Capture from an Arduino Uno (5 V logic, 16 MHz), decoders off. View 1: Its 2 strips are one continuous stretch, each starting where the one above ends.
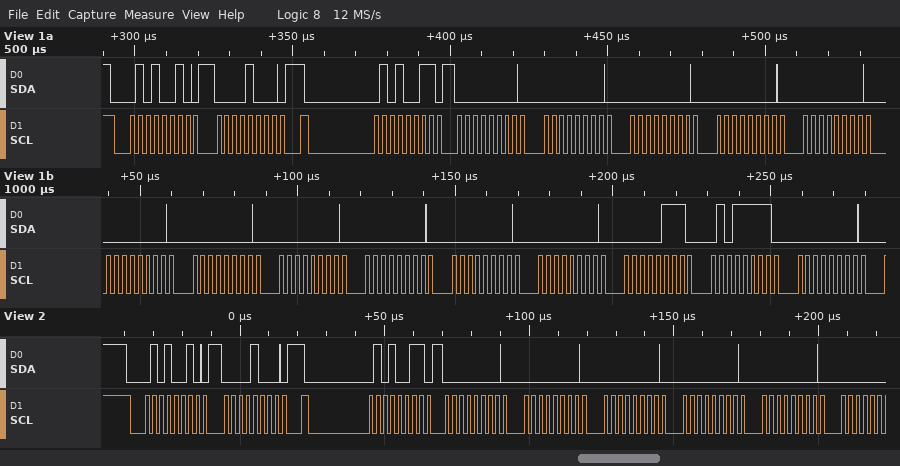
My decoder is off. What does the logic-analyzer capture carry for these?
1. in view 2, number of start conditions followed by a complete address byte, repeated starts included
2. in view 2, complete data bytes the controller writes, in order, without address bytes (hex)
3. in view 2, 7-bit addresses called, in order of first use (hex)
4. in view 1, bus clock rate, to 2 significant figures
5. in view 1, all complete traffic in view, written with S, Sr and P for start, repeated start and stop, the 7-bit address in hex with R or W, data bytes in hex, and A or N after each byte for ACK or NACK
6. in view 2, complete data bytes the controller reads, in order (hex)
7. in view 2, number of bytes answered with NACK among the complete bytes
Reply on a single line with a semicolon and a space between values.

2; 08; 0x29; 400 kHz; S 29W A 08 A Sr 29R A 00 A 00 A 00 A 00 A 00 A 00 A 00 A 00 A 00 A 00 A 00 A 07 A 5F A 00 A; 00 00 00 00 00; 0
